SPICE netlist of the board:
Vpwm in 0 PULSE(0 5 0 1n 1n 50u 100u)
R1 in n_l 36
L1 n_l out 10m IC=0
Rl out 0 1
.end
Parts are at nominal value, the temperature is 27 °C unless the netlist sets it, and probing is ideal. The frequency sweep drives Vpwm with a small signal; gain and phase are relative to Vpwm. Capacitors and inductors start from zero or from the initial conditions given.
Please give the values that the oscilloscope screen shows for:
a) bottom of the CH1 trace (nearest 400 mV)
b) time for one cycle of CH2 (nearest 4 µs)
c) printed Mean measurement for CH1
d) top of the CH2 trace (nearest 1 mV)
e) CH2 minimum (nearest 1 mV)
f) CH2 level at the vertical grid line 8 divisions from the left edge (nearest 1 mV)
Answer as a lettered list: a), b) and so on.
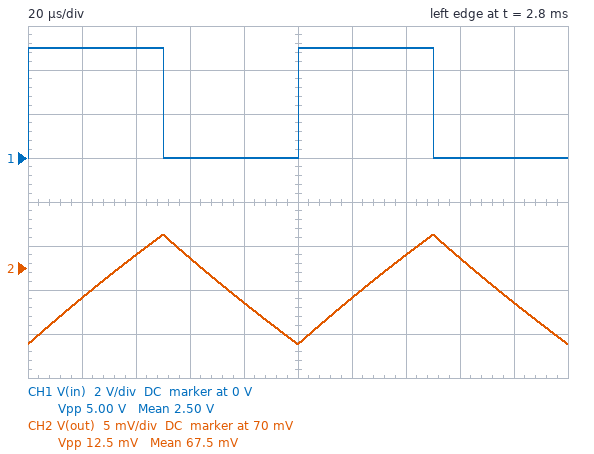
a) 0 V
b) 100 µs
c) 2.50 V
d) 74 mV
e) 61 mV
f) 71 mV
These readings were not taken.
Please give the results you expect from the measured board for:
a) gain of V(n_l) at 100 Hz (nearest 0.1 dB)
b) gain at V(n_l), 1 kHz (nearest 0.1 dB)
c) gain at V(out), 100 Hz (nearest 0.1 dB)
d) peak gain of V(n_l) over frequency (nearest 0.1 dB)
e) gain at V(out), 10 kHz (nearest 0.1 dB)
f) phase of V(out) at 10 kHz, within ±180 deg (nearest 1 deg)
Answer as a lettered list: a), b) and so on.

a) -15.4 dB
b) -1.3 dB
c) -31.5 dB
d) 0 dB
e) -56.0 dB
f) -87 deg
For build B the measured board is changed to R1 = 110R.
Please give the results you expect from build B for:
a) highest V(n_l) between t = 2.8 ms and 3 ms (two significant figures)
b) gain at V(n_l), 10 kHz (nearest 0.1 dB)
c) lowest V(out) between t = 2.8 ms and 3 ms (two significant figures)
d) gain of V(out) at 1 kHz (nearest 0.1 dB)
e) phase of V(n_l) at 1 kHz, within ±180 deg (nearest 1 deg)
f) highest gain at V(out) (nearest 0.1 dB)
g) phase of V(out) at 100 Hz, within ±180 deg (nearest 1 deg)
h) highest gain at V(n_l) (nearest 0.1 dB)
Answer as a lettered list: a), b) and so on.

a) 3.2 V
b) -0.1 dB
c) 16 mV
d) -42.1 dB
e) 60 deg
f) -40.9 dB
g) -3 deg
h) 0 dB
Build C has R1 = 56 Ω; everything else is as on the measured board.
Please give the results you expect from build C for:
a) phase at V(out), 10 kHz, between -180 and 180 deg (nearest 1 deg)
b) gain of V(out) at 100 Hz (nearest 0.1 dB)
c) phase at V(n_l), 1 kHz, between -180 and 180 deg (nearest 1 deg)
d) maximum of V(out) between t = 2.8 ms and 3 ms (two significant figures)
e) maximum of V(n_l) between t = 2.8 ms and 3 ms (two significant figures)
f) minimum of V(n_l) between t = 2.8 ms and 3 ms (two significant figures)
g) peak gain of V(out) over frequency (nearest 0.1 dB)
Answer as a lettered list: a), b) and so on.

a) -85 deg
b) -35.2 dB
c) 41 deg
d) 50 mV
e) 2.9 V
f) -2.8 V
g) -35.1 dB
